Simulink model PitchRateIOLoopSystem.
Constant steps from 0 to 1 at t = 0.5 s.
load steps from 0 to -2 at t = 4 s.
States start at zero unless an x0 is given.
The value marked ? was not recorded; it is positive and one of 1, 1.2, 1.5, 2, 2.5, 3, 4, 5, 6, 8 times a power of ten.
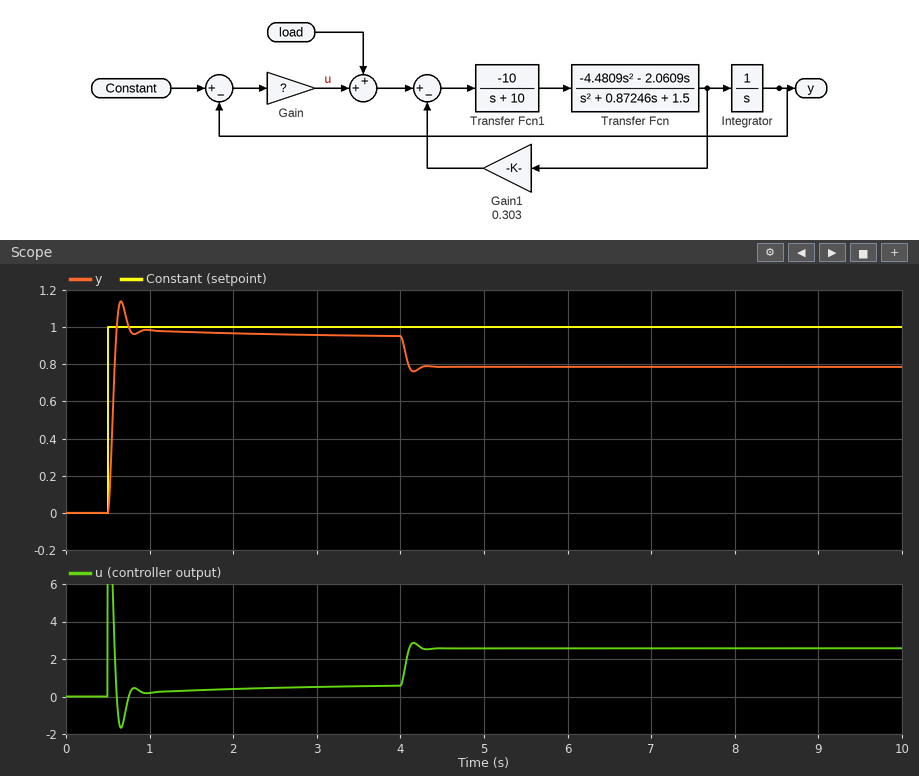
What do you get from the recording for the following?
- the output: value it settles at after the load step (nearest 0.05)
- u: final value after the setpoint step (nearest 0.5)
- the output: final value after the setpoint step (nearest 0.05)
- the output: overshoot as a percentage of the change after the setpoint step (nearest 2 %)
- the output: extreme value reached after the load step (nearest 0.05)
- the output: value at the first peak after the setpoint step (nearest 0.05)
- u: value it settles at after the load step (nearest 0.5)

0.80
0.5
0.95
20 %
0.75
1.15
2.5
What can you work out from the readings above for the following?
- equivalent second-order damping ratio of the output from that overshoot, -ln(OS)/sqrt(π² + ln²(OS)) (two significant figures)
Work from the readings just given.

0.46
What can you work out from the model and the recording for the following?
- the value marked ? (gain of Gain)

12
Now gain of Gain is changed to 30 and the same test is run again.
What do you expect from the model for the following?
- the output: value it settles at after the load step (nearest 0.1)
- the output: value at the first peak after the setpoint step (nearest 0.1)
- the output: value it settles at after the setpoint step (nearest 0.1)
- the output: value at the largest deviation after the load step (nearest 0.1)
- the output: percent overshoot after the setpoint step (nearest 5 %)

0.9
1.3
1.0
0.9
35 %
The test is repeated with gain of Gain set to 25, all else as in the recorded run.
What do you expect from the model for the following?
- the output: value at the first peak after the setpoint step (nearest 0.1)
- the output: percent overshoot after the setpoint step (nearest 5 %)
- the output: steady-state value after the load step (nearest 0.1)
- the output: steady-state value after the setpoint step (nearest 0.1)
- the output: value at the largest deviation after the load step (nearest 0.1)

1.3
35 %
0.9
1.0
0.9
